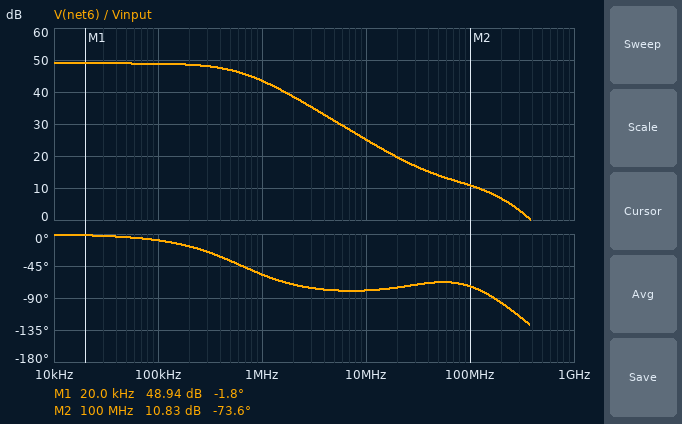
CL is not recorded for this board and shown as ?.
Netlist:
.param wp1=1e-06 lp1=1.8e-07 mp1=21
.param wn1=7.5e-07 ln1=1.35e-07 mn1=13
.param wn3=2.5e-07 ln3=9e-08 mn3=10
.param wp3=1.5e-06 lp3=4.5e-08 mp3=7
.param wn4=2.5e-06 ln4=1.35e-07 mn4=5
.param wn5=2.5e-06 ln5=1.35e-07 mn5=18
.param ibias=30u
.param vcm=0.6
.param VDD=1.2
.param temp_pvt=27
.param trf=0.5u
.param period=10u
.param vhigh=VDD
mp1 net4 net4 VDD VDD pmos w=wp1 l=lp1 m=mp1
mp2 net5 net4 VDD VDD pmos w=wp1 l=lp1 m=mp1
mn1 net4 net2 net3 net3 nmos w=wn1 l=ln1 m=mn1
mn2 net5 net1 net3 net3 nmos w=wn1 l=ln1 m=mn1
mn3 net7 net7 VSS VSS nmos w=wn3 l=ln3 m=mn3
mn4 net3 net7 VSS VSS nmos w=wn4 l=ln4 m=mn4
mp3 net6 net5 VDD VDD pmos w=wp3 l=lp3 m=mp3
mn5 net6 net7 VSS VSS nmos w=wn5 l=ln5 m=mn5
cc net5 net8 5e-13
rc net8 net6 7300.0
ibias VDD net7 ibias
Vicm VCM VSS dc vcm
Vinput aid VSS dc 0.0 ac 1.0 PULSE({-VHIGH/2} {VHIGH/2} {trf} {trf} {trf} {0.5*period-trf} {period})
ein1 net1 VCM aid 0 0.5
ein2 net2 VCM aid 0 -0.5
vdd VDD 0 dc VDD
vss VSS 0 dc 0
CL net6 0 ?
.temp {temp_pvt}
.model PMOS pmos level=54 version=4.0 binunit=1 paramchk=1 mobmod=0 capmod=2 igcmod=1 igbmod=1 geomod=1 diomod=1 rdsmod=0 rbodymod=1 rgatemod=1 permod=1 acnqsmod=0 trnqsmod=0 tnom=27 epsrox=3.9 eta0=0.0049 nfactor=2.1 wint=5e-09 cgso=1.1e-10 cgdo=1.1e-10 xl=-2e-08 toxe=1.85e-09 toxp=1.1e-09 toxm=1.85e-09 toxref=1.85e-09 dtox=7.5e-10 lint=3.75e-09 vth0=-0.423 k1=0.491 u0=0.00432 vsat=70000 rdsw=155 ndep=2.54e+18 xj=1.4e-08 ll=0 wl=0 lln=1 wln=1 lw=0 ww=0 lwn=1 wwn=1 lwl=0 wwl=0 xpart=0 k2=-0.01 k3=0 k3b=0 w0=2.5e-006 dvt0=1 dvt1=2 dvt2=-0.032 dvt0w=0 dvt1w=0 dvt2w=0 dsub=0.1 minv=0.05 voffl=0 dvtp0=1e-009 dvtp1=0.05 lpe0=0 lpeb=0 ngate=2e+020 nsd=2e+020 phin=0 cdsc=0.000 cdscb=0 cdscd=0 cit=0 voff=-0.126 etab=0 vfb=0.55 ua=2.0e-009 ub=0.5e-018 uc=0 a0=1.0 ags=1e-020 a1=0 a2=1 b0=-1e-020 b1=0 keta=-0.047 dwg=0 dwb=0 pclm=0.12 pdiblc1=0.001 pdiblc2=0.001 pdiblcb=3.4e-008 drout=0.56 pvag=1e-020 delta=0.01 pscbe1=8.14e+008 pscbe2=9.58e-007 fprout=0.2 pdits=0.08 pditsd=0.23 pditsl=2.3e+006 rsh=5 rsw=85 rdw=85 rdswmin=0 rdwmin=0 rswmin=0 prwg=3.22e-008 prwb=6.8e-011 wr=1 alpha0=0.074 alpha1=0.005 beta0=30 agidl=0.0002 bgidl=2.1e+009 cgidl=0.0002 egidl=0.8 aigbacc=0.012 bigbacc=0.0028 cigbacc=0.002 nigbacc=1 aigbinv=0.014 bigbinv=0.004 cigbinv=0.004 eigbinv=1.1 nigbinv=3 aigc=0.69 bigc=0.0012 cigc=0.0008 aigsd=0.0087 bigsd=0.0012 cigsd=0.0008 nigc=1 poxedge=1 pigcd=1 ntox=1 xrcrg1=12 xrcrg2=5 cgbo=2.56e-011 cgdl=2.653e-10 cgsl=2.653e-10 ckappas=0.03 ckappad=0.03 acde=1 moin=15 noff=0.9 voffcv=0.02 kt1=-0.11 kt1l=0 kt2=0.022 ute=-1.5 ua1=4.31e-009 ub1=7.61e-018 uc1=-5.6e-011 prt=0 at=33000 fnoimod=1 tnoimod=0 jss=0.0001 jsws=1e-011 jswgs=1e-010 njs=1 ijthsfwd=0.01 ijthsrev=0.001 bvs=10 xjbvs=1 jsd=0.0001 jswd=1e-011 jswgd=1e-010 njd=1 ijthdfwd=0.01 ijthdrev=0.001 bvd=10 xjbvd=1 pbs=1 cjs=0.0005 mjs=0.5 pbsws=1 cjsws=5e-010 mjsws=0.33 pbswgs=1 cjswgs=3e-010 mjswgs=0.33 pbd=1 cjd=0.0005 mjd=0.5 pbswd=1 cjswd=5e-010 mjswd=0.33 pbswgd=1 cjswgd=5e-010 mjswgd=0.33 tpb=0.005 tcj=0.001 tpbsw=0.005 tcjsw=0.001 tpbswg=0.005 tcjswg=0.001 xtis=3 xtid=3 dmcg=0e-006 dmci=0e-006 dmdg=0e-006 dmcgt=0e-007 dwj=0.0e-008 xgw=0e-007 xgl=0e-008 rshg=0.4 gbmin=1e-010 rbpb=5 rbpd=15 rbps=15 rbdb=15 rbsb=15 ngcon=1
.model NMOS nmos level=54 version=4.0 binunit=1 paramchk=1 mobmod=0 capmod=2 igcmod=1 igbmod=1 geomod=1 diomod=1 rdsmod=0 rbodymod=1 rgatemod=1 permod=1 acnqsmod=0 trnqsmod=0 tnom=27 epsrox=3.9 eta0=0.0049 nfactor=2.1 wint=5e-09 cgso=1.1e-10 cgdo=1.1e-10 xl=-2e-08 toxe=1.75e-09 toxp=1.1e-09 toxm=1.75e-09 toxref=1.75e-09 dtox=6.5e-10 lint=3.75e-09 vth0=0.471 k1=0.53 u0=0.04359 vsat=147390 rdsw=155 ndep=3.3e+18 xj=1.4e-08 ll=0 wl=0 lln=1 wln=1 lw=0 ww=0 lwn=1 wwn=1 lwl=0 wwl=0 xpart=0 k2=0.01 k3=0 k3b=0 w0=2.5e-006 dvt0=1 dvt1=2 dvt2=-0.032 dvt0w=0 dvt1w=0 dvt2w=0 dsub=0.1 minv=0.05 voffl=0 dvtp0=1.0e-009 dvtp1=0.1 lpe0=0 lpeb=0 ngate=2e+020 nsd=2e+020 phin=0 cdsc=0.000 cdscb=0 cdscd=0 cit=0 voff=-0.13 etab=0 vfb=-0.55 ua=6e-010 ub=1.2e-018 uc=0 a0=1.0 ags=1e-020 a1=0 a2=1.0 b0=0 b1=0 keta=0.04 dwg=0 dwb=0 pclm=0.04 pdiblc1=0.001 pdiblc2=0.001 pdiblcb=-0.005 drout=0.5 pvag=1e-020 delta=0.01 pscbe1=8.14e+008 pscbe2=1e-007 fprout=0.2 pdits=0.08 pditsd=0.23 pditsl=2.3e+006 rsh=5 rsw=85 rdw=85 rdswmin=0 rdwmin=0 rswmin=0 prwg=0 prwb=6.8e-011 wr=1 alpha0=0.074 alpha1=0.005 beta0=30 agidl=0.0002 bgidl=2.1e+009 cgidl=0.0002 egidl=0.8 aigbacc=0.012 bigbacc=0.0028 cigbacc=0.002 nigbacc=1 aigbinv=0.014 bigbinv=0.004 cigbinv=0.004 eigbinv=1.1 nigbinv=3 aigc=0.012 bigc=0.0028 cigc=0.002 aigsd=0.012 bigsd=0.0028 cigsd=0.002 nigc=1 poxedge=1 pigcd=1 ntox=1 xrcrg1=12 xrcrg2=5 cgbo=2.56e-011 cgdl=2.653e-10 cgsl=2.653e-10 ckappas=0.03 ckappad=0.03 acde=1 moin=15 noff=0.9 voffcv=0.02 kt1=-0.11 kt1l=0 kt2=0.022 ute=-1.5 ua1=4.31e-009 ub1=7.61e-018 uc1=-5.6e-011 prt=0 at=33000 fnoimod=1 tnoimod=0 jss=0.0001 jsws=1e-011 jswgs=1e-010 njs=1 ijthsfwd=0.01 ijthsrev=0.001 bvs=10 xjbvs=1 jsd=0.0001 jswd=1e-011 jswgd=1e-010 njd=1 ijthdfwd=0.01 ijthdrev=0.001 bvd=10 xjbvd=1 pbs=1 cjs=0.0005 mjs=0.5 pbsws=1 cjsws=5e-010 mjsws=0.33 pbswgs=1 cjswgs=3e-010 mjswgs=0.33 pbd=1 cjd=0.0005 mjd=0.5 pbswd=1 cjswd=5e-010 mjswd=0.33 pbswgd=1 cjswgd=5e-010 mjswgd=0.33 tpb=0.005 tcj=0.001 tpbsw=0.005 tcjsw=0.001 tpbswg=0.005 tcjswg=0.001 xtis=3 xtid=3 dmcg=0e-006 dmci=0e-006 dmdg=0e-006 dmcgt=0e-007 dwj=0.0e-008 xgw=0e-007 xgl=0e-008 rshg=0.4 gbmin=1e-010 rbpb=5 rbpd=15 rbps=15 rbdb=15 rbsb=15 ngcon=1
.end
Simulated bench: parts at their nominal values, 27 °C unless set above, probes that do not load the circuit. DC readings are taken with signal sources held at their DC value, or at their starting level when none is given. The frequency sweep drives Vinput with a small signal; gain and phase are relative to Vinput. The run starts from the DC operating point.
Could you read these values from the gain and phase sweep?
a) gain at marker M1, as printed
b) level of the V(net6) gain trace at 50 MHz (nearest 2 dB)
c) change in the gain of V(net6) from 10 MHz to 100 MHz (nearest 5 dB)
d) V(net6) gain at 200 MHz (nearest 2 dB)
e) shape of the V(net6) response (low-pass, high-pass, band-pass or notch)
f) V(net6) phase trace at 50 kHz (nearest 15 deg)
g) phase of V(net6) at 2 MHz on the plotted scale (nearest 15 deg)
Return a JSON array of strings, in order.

["48.94 dB", "14 dB", "-15 dB", "6 dB", "low-pass", "0 deg", "-75 deg"]
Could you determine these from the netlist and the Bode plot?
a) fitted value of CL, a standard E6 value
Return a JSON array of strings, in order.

["4.7 pF"]
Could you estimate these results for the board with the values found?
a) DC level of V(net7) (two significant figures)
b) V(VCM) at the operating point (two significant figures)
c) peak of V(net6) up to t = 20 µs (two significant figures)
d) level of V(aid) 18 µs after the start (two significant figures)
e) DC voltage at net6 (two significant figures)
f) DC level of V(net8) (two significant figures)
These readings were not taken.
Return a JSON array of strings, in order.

["460 mV", "600 mV", "1.2 V", "-600 mV", "960 mV", "960 mV"]
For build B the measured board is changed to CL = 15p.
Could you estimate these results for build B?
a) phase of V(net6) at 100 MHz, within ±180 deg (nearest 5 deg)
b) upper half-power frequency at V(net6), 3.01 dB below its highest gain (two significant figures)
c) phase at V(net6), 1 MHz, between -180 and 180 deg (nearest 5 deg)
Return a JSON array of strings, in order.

["-105 deg", "610 kHz", "-60 deg"]
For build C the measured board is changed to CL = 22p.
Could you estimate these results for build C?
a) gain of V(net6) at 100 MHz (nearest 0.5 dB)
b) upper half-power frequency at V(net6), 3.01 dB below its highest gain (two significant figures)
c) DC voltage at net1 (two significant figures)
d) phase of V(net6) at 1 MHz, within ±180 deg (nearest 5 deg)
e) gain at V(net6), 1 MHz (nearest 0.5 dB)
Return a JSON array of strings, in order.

["1.0 dB", "600 kHz", "600 mV", "-60 deg", "43.0 dB"]
